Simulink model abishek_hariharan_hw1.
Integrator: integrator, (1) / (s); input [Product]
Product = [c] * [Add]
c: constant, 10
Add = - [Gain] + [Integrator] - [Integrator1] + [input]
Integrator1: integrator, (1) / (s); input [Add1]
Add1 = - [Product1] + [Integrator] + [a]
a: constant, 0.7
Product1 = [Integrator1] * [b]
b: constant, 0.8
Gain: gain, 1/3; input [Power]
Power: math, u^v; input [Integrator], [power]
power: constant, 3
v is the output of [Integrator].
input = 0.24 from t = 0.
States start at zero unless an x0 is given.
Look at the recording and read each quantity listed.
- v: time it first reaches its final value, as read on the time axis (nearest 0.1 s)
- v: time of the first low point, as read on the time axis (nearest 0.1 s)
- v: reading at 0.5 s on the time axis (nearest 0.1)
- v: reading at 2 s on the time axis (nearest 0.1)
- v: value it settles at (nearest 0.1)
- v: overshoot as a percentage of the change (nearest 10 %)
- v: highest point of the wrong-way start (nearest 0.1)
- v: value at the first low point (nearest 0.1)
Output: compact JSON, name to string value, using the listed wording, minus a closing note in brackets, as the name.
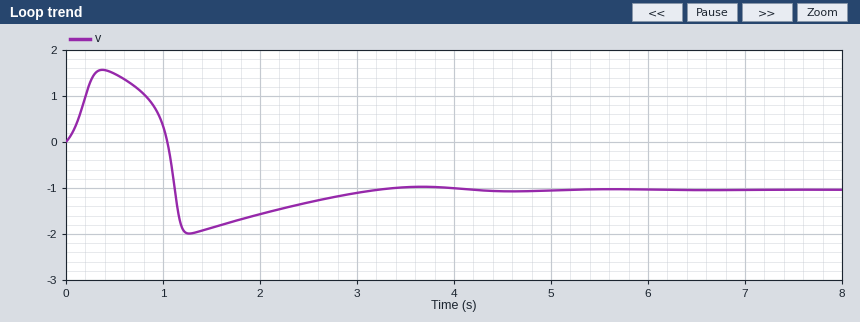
{"v: time it first reaches its final value, as read on the time axis": "1.1 s", "v: time of the first low point, as read on the time axis": "1.3 s", "v: reading at 0.5 s on the time axis": "1.5", "v: reading at 2 s on the time axis": "-1.6", "v: value it settles at": "-1.0", "v: overshoot as a percentage of the change": "90 %", "v: highest point of the wrong-way start": "1.6", "v: value at the first low point": "-2.0"}
